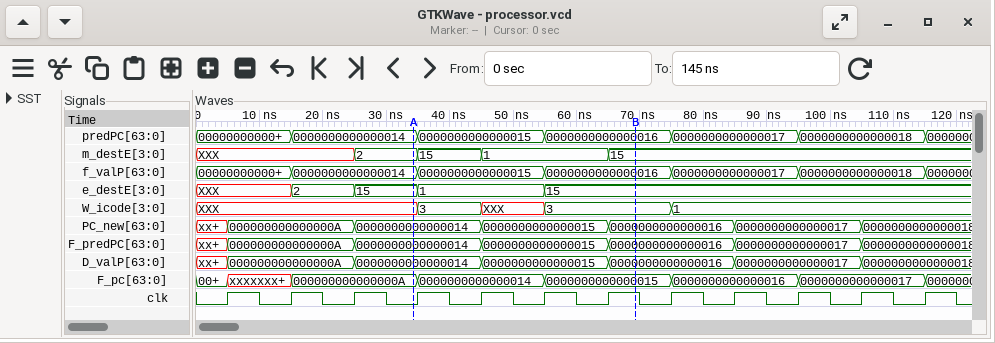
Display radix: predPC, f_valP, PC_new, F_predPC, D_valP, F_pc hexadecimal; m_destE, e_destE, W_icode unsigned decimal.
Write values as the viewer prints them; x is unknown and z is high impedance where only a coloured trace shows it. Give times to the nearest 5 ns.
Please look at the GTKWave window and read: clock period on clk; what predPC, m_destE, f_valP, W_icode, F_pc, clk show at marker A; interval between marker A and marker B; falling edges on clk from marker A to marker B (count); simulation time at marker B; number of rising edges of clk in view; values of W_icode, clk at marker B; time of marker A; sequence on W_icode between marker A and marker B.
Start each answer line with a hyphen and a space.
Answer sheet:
- 10 ns
- predPC=0000000000000014, m_destE=2, f_valP=0000000000000014, W_icode=XXX, F_pc=000000000000000A, clk=0
- 35 ns
- 3
- 70 ns
- 12
- W_icode=3, clk=1
- 35 ns
- XXX, 3, XXX, 3
